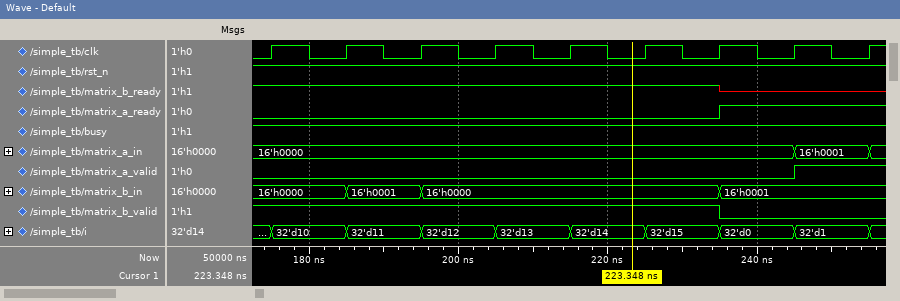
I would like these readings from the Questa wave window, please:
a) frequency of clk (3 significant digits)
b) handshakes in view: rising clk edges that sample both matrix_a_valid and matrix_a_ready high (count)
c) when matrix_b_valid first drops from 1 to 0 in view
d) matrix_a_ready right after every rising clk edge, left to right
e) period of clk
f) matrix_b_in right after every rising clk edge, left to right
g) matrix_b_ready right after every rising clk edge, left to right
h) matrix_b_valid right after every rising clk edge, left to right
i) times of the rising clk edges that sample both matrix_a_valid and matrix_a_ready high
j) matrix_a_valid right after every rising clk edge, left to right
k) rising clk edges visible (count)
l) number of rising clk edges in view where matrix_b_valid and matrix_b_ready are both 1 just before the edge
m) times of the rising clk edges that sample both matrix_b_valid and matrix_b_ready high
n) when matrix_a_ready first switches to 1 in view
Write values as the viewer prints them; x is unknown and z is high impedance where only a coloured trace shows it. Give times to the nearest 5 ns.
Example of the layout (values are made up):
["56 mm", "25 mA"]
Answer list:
["100 MHz", "1", "235 ns", "0 0 0 0 0 0 1 1 1", "10 ns", "16'h0000, 16'h0001, 16'h0000, 16'h0000, 16'h0000, 16'h0000, 16'h0001, 16'h0001, 16'h0001", "1 1 1 1 1 1 x x x", "1 1 1 1 1 1 0 0 0", "255 ns", "0 0 0 0 0 0 0 1 1", "9", "7", "175 ns, 185 ns, 195 ns, 205 ns, 215 ns, 225 ns, 235 ns", "235 ns"]
